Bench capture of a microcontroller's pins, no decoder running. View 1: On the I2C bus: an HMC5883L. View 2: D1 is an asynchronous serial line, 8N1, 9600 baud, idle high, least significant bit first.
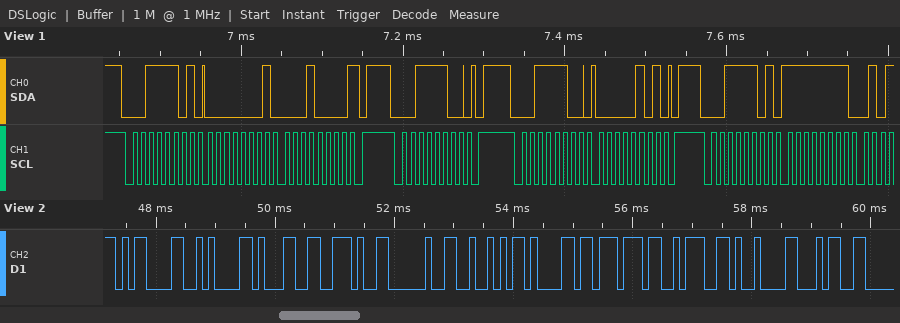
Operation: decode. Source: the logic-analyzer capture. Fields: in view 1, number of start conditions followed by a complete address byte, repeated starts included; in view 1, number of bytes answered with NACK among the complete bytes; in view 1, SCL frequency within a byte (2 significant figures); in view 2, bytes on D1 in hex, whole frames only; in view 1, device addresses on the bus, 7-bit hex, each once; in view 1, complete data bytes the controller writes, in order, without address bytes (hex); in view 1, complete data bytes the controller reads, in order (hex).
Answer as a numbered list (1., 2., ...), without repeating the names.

1. 4
2. 1
3. 100 kHz
4. 0D 0A 31 2E 20 52 61 77 3A 09 34
5. 0x1E
6. 05
7. 01 10 FF
